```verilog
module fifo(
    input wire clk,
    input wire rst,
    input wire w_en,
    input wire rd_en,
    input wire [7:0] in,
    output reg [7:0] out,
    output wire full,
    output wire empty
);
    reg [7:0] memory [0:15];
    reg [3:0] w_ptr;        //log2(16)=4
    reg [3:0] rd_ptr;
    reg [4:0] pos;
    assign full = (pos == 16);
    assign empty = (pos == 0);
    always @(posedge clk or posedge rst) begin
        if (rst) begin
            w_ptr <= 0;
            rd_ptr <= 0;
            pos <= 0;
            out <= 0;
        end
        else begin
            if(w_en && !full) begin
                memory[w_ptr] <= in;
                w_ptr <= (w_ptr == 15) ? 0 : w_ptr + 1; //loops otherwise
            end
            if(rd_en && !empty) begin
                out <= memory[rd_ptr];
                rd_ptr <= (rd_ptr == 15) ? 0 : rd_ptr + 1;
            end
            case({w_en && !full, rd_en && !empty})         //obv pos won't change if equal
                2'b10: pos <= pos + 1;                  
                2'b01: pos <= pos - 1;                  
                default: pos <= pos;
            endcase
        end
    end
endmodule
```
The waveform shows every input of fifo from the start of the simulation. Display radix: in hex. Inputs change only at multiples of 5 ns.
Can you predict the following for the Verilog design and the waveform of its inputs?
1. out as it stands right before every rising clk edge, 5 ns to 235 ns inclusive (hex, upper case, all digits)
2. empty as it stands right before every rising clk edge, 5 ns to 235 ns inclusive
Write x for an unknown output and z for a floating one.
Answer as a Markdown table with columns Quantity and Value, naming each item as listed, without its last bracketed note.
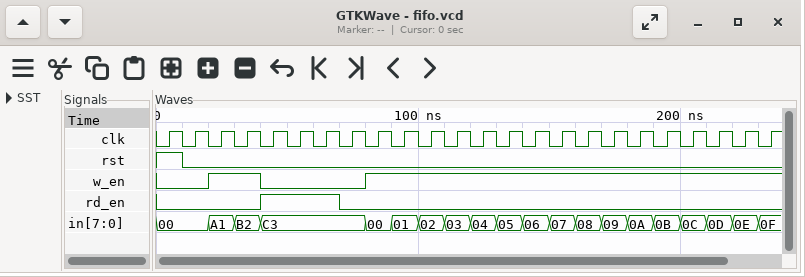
| Quantity | Value |
|---|---|
| out as it stands right before every rising clk edge, 5 ns to 235 ns inclusive | 00, 00, 00, 00, 00, A1, B2, B2, B2, B2, B2, B2, B2, B2, B2, B2, B2, B2, B2, B2, B2, B2, B2, B2 |
| empty as it stands right before every rising clk edge, 5 ns to 235 ns inclusive | 1 1 1 0 0 0 1 1 1 0 0 0 0 0 0 0 0 0 0 0 0 0 0 0 |
